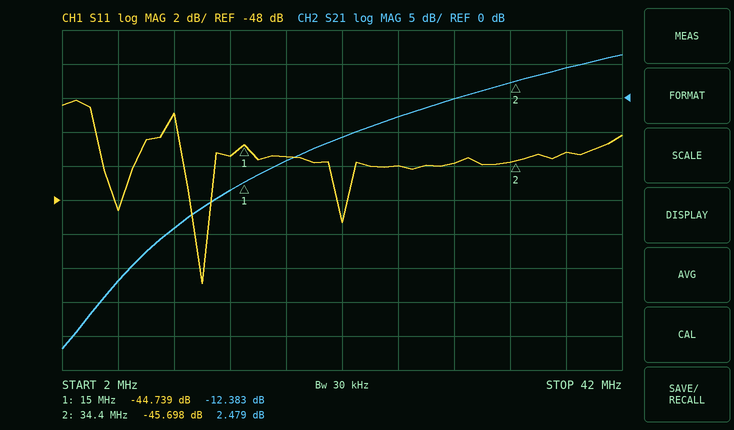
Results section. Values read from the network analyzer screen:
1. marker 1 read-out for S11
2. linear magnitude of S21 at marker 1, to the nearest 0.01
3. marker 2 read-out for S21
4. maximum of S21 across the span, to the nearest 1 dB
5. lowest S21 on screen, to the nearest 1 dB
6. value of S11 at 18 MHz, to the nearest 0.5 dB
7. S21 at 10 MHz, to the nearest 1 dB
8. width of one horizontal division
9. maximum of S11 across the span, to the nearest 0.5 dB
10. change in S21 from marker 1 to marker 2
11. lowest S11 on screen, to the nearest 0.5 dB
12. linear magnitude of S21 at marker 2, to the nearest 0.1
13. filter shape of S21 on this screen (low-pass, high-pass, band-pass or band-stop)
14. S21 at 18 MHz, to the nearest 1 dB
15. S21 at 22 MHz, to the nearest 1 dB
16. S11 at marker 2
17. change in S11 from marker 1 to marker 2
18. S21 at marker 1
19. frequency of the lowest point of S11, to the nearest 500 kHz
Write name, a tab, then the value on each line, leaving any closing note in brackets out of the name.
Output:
marker 1 read-out for S11	-44.739 dB
linear magnitude of S21 at marker 1, to the nearest 0.01	0.24
marker 2 read-out for S21	2.479 dB
maximum of S21 across the span, to the nearest 1 dB	6 dB
lowest S21 on screen, to the nearest 1 dB	-37 dB
value of S11 at 18 MHz, to the nearest 0.5 dB	-45.5 dB
S21 at 10 MHz, to the nearest 1 dB	-19 dB
width of one horizontal division	4 MHz
maximum of S11 across the span, to the nearest 0.5 dB	-42.0 dB
change in S21 from marker 1 to marker 2	14.862 dB
lowest S11 on screen, to the nearest 0.5 dB	-53.0 dB
linear magnitude of S21 at marker 2, to the nearest 0.1	1.3
filter shape of S21 on this screen	high-pass
S21 at 18 MHz, to the nearest 1 dB	-9 dB
S21 at 22 MHz, to the nearest 1 dB	-6 dB
S11 at marker 2	-45.698 dB
change in S11 from marker 1 to marker 2	-0.959 dB
S21 at marker 1	-12.383 dB
frequency of the lowest point of S11, to the nearest 500 kHz	12.0 MHz
